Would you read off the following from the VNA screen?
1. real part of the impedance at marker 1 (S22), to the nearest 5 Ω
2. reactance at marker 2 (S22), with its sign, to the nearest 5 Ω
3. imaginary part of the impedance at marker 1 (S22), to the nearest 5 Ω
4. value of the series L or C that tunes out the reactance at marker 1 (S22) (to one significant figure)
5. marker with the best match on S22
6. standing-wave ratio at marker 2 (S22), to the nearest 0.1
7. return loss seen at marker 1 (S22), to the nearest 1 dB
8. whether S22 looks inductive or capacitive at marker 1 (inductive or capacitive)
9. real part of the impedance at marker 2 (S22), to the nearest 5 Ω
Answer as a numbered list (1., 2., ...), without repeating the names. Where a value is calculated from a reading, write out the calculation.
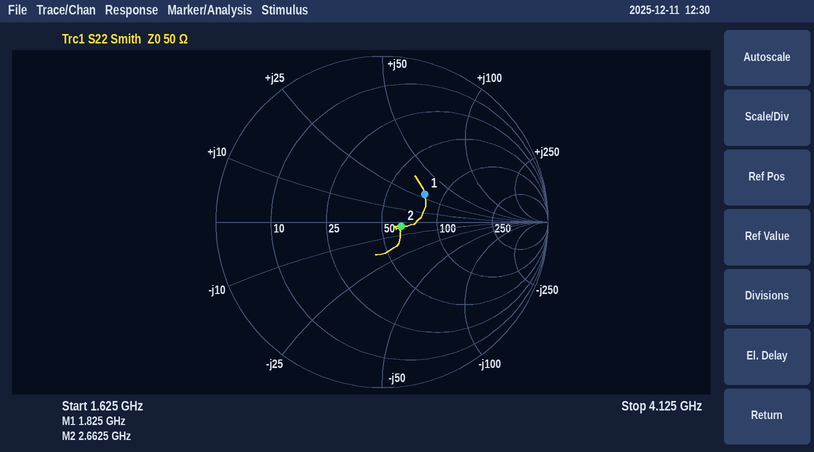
1. 80 Ω
2. -5 Ω
3. +30 Ω
4. C = 1/(2π × 1.825 GHz × 30 Ω) ≈ 3 pF
5. marker 2
6. 1.3
7. 10 dB
8. inductive
9. 65 Ω
